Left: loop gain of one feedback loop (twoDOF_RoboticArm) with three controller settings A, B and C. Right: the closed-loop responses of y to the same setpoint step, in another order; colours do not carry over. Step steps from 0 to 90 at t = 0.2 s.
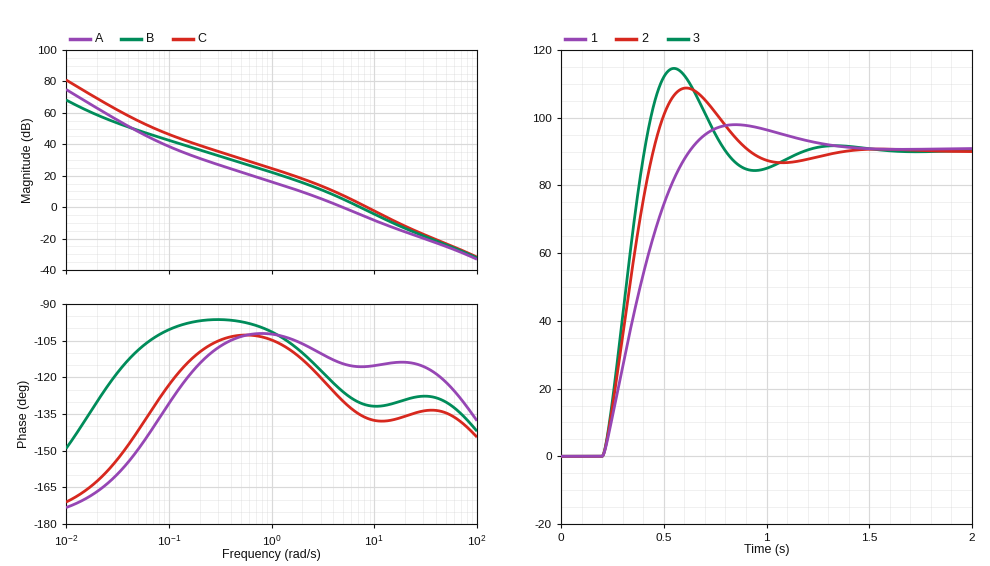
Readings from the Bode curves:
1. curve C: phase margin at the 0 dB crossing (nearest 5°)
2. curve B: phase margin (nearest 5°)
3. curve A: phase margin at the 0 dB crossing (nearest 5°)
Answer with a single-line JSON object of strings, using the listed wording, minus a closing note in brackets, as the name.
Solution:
{"curve C: phase margin at the 0 dB crossing": "45°", "curve B: phase margin": "50°", "curve A: phase margin at the 0 dB crossing": "65°"}
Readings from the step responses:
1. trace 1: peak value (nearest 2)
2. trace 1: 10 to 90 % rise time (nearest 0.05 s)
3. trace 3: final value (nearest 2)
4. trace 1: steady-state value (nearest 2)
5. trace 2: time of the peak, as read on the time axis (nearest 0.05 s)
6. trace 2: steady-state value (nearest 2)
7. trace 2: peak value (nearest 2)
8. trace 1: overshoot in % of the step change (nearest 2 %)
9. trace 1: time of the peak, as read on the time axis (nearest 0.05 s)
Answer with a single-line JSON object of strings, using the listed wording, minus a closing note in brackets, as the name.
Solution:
{"trace 1: peak value": "98", "trace 1: 10 to 90 % rise time": "0.30 s", "trace 3: final value": "90", "trace 1: steady-state value": "90", "trace 2: time of the peak, as read on the time axis": "0.60 s", "trace 2: steady-state value": "90", "trace 2: peak value": "108", "trace 1: overshoot in % of the step change": "8 %", "trace 1: time of the peak, as read on the time axis": "0.85 s"}
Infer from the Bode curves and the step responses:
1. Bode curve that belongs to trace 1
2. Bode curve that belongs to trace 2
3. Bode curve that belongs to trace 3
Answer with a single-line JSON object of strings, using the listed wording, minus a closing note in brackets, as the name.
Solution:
{"Bode curve that belongs to trace 1": "A", "Bode curve that belongs to trace 2": "B", "Bode curve that belongs to trace 3": "C"}
